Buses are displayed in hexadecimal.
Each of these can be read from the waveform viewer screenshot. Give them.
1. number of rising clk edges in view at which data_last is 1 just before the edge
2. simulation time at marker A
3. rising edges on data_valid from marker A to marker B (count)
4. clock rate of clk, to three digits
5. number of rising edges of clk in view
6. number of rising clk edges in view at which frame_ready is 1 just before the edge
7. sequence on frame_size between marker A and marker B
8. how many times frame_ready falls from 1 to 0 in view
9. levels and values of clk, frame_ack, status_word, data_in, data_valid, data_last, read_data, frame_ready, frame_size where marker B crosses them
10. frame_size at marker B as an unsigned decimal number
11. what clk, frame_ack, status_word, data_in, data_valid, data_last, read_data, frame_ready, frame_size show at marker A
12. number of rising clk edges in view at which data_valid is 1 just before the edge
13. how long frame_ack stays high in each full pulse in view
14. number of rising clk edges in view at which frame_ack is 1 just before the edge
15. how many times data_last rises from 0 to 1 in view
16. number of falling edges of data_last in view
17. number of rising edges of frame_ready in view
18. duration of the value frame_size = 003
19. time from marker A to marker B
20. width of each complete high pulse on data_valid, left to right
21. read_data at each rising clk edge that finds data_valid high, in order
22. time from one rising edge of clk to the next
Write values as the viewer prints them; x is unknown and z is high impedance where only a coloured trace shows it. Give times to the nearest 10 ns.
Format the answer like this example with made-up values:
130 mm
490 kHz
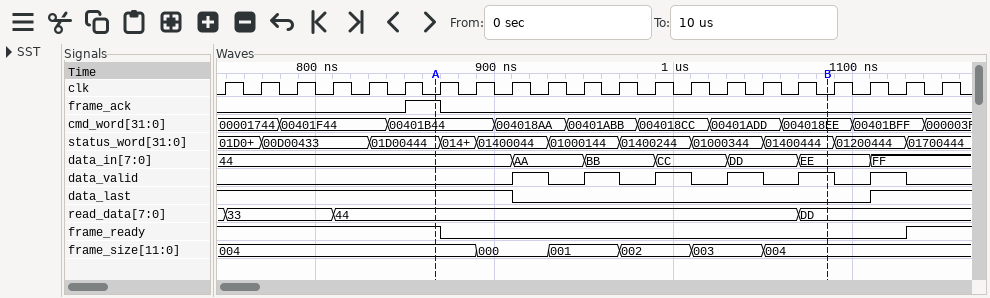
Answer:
11
870 ns
5
50.0 MHz
21
8
004, 000, 001, 002, 003, 004
1
clk=0, frame_ack=0, status_word=01400444, data_in=EE, data_valid=1, data_last=0, read_data=DD, frame_ready=0, frame_size=004
4
clk=0, frame_ack=1, status_word=01D00444, data_in=44, data_valid=0, data_last=1, read_data=44, frame_ready=1, frame_size=004
6
20 ns
1
1
1
1
40 ns
220 ns
20 ns, 20 ns, 20 ns, 20 ns, 20 ns, 20 ns
44, 44, 44, 44, DD, DD
20 ns
